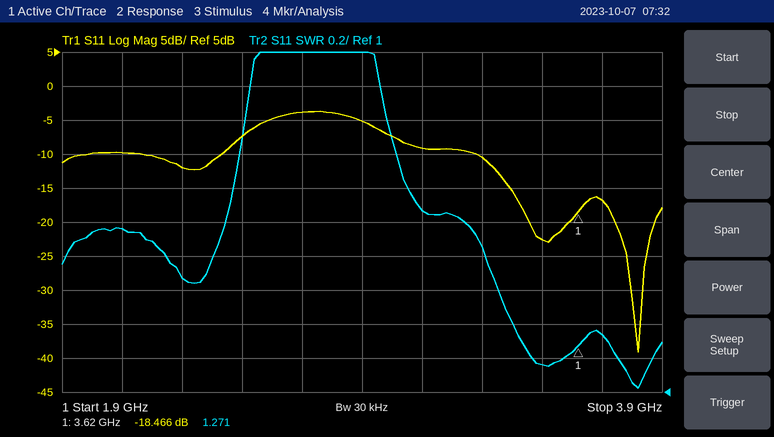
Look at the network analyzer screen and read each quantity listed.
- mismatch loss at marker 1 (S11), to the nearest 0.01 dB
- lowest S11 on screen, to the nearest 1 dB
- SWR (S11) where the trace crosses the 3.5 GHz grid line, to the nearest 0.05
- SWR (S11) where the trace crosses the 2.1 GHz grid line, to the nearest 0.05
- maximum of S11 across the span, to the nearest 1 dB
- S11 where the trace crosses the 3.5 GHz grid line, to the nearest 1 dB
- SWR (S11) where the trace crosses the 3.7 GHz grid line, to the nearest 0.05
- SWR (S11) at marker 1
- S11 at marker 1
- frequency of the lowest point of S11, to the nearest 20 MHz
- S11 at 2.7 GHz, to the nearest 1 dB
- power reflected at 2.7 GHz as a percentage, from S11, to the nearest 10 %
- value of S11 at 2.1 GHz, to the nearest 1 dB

0.06 dB
-39 dB
1.15
1.95
-4 dB
-23 dB
1.35
1.271
-18.466 dB
3.82 GHz
-4 dB
40 %
-10 dB
